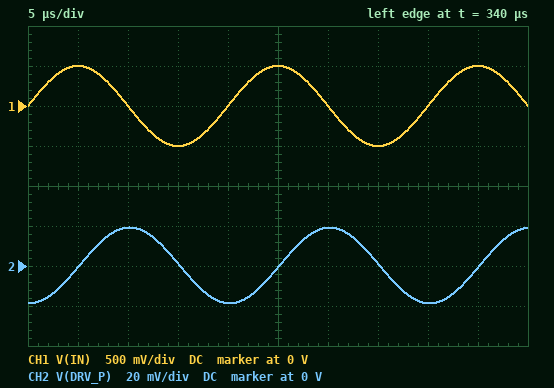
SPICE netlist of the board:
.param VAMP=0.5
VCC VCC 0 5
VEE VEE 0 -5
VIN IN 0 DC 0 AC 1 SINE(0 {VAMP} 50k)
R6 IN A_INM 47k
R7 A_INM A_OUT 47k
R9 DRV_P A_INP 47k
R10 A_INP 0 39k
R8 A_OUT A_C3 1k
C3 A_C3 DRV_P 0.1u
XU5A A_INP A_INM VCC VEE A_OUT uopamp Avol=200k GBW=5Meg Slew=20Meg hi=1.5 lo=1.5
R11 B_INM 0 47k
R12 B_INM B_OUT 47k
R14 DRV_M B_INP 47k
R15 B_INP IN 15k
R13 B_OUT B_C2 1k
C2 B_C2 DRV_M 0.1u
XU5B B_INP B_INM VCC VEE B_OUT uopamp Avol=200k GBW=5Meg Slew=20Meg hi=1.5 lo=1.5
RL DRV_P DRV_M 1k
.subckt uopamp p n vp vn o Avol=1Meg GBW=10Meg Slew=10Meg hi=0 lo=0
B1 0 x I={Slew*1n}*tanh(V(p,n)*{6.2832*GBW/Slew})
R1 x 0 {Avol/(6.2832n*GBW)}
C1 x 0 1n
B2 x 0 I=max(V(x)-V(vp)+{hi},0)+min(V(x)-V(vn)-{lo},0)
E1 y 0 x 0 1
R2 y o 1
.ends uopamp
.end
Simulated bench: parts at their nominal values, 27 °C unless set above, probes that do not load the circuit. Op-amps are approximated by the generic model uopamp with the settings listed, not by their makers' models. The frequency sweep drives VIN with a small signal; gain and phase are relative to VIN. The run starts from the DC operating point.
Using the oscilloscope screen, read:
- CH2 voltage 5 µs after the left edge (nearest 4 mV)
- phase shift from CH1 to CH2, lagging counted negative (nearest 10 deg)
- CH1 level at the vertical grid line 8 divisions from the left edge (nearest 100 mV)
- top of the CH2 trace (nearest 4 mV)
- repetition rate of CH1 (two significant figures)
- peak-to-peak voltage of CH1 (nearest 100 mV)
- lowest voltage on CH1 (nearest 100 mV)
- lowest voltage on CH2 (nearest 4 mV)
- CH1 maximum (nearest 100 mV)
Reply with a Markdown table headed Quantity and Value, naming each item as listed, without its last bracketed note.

| Quantity | Value |
|---|---|
| CH2 voltage 5 µs after the left edge | 0 V |
| phase shift from CH1 to CH2, lagging counted negative | -90 deg |
| CH1 level at the vertical grid line 8 divisions from the left edge | 0 V |
| top of the CH2 trace | 20 mV |
| repetition rate of CH1 | 50 kHz |
| peak-to-peak voltage of CH1 | 1.0 V |
| lowest voltage on CH1 | -500 mV |
| lowest voltage on CH2 | -20 mV |
| CH1 maximum | 500 mV |
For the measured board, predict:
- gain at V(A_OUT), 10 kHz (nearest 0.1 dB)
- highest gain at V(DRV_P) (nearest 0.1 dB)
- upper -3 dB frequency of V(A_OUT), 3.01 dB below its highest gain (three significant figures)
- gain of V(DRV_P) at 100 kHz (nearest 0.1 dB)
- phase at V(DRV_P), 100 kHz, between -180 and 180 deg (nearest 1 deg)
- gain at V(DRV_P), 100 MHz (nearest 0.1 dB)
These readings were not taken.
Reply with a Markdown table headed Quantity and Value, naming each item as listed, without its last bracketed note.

| Quantity | Value |
|---|---|
| gain at V(A_OUT), 10 kHz | -0.1 dB |
| highest gain at V(DRV_P) | -1.9 dB |
| upper -3 dB frequency of V(A_OUT), 3.01 dB below its highest gain | 2.58 MHz |
| gain of V(DRV_P) at 100 kHz | -28.2 dB |
| phase at V(DRV_P), 100 kHz, between -180 and 180 deg | -99 deg |
| gain at V(DRV_P), 100 MHz | -43.7 dB |
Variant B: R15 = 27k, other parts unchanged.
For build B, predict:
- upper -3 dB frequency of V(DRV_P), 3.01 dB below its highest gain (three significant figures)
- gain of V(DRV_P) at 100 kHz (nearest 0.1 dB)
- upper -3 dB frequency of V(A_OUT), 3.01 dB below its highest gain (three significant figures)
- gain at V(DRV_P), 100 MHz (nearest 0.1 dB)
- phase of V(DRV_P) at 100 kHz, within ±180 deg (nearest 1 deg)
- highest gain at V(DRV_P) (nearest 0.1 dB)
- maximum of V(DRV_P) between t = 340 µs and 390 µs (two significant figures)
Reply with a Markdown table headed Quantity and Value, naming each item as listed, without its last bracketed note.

| Quantity | Value |
|---|---|
| upper -3 dB frequency of V(DRV_P), 3.01 dB below its highest gain | 1.62 kHz |
| gain of V(DRV_P) at 100 kHz | -22.2 dB |
| upper -3 dB frequency of V(A_OUT), 3.01 dB below its highest gain | 2.33 MHz |
| gain at V(DRV_P), 100 MHz | -42.7 dB |
| phase of V(DRV_P) at 100 kHz, within ±180 deg | -104 deg |
| highest gain at V(DRV_P) | -3.2 dB |
| maximum of V(DRV_P) between t = 340 µs and 390 µs | 28 mV |
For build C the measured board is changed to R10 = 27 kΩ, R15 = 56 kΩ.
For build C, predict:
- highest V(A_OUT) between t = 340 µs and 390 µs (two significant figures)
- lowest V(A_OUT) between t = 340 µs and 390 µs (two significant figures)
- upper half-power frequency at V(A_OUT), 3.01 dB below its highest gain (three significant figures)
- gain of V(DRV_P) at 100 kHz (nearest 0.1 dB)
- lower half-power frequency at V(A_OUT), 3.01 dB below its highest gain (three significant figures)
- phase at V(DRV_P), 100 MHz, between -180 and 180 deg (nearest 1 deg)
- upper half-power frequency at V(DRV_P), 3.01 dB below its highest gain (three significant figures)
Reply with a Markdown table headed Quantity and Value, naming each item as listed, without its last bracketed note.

| Quantity | Value |
|---|---|
| highest V(A_OUT) between t = 340 µs and 390 µs | 510 mV |
| lowest V(A_OUT) between t = 340 µs and 390 µs | -510 mV |
| upper half-power frequency at V(A_OUT), 3.01 dB below its highest gain | 2.05 MHz |
| gain of V(DRV_P) at 100 kHz | -13.7 dB |
| lower half-power frequency at V(A_OUT), 3.01 dB below its highest gain | 111 Hz |
| phase at V(DRV_P), 100 MHz, between -180 and 180 deg | 71 deg |
| upper half-power frequency at V(DRV_P), 3.01 dB below its highest gain | 2.17 MHz |
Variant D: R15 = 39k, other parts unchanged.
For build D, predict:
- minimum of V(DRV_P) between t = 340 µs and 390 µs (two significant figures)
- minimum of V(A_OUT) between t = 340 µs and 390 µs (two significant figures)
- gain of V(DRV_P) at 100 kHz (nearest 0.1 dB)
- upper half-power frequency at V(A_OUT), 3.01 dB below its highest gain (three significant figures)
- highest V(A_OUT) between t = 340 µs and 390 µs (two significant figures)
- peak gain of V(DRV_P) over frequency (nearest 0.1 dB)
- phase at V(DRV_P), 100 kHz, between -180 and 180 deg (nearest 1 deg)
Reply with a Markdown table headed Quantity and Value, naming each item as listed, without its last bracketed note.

| Quantity | Value |
|---|---|
| minimum of V(DRV_P) between t = 340 µs and 390 µs | -47 mV |
| minimum of V(A_OUT) between t = 340 µs and 390 µs | -510 mV |
| gain of V(DRV_P) at 100 kHz | -16.0 dB |
| upper half-power frequency at V(A_OUT), 3.01 dB below its highest gain | 2.07 MHz |
| highest V(A_OUT) between t = 340 µs and 390 µs | 510 mV |
| peak gain of V(DRV_P) over frequency | -6.1 dB |
| phase at V(DRV_P), 100 kHz, between -180 and 180 deg | -113 deg |
